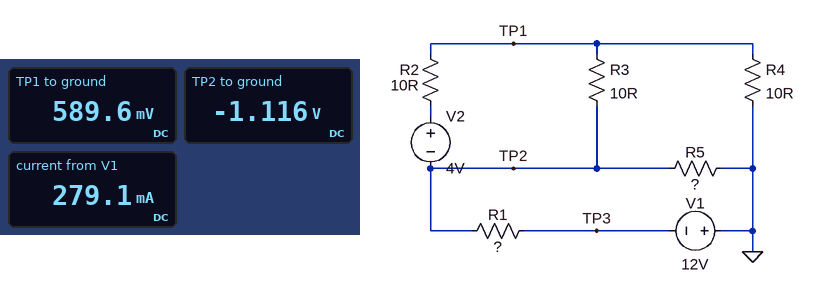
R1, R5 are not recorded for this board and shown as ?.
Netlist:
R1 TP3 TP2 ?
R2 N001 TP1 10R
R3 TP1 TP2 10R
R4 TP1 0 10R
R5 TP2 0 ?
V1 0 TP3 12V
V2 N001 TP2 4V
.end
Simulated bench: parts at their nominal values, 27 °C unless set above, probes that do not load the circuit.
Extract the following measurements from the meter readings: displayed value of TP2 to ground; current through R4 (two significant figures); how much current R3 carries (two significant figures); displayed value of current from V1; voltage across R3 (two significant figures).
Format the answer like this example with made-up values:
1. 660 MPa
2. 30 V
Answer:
1. -1.116 V
2. 59 mA
3. 170 mA
4. 279.1 mA
5. 1.7 V
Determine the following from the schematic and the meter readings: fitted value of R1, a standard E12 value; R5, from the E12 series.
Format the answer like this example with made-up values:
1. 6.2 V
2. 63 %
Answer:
1. 39 Ω
2. 3.3 Ω
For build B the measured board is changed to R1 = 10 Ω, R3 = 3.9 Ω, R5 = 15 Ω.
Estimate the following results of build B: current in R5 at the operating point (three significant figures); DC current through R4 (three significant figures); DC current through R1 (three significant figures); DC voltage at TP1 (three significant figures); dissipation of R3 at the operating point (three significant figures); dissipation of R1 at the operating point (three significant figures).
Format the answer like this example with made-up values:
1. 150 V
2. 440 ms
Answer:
1. 351 mA
2. 323 mA
3. 674 mA
4. -3.23 V
5. 1.06 W
6. 4.54 W
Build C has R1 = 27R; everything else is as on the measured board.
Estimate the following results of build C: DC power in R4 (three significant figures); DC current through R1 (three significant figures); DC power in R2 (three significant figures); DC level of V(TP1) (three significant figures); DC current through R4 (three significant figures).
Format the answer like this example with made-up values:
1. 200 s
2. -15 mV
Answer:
1. 14.9 mW
2. 392 mA
3. 481 mW
4. 386 mV
5. 38.6 mA
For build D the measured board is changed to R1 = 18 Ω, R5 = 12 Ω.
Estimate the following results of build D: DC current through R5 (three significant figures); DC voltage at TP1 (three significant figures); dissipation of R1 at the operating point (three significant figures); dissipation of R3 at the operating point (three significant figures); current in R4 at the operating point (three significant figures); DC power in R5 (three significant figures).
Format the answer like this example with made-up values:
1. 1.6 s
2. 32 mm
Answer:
1. 324 mA
2. -1.26 V
3. 3.65 W
4. 692 mW
5. 126 mA
6. 1.26 W
